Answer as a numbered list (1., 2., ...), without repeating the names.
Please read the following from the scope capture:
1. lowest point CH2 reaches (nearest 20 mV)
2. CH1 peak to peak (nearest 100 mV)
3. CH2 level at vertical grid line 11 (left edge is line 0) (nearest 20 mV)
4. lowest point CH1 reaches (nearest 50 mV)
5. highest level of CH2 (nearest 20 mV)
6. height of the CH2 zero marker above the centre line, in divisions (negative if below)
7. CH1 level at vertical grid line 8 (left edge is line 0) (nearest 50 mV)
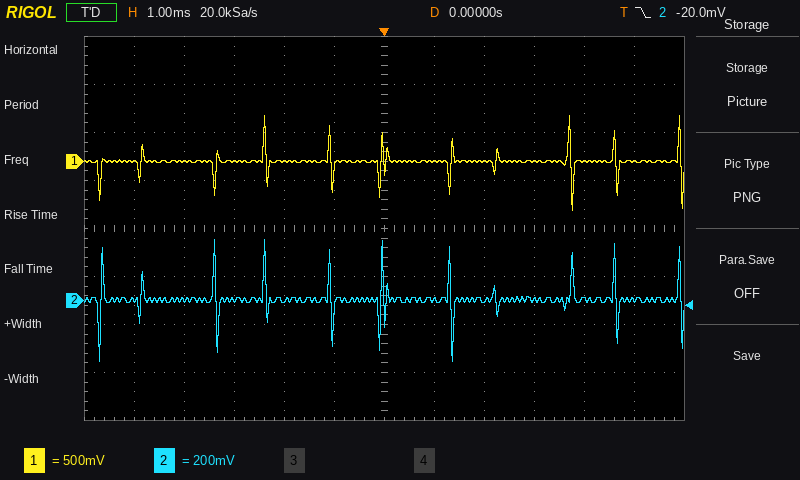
1. -260 mV
2. 1.00 V
3. 0 mV
4. -500 mV
5. 260 mV
6. -1.5 div
7. 0 mV
